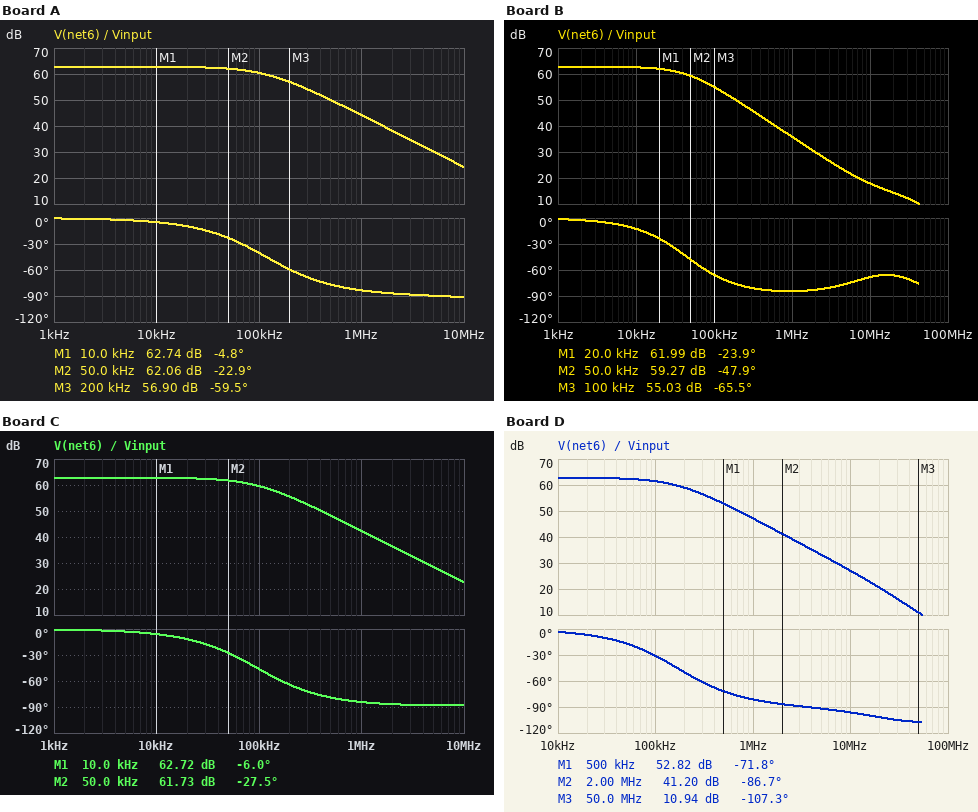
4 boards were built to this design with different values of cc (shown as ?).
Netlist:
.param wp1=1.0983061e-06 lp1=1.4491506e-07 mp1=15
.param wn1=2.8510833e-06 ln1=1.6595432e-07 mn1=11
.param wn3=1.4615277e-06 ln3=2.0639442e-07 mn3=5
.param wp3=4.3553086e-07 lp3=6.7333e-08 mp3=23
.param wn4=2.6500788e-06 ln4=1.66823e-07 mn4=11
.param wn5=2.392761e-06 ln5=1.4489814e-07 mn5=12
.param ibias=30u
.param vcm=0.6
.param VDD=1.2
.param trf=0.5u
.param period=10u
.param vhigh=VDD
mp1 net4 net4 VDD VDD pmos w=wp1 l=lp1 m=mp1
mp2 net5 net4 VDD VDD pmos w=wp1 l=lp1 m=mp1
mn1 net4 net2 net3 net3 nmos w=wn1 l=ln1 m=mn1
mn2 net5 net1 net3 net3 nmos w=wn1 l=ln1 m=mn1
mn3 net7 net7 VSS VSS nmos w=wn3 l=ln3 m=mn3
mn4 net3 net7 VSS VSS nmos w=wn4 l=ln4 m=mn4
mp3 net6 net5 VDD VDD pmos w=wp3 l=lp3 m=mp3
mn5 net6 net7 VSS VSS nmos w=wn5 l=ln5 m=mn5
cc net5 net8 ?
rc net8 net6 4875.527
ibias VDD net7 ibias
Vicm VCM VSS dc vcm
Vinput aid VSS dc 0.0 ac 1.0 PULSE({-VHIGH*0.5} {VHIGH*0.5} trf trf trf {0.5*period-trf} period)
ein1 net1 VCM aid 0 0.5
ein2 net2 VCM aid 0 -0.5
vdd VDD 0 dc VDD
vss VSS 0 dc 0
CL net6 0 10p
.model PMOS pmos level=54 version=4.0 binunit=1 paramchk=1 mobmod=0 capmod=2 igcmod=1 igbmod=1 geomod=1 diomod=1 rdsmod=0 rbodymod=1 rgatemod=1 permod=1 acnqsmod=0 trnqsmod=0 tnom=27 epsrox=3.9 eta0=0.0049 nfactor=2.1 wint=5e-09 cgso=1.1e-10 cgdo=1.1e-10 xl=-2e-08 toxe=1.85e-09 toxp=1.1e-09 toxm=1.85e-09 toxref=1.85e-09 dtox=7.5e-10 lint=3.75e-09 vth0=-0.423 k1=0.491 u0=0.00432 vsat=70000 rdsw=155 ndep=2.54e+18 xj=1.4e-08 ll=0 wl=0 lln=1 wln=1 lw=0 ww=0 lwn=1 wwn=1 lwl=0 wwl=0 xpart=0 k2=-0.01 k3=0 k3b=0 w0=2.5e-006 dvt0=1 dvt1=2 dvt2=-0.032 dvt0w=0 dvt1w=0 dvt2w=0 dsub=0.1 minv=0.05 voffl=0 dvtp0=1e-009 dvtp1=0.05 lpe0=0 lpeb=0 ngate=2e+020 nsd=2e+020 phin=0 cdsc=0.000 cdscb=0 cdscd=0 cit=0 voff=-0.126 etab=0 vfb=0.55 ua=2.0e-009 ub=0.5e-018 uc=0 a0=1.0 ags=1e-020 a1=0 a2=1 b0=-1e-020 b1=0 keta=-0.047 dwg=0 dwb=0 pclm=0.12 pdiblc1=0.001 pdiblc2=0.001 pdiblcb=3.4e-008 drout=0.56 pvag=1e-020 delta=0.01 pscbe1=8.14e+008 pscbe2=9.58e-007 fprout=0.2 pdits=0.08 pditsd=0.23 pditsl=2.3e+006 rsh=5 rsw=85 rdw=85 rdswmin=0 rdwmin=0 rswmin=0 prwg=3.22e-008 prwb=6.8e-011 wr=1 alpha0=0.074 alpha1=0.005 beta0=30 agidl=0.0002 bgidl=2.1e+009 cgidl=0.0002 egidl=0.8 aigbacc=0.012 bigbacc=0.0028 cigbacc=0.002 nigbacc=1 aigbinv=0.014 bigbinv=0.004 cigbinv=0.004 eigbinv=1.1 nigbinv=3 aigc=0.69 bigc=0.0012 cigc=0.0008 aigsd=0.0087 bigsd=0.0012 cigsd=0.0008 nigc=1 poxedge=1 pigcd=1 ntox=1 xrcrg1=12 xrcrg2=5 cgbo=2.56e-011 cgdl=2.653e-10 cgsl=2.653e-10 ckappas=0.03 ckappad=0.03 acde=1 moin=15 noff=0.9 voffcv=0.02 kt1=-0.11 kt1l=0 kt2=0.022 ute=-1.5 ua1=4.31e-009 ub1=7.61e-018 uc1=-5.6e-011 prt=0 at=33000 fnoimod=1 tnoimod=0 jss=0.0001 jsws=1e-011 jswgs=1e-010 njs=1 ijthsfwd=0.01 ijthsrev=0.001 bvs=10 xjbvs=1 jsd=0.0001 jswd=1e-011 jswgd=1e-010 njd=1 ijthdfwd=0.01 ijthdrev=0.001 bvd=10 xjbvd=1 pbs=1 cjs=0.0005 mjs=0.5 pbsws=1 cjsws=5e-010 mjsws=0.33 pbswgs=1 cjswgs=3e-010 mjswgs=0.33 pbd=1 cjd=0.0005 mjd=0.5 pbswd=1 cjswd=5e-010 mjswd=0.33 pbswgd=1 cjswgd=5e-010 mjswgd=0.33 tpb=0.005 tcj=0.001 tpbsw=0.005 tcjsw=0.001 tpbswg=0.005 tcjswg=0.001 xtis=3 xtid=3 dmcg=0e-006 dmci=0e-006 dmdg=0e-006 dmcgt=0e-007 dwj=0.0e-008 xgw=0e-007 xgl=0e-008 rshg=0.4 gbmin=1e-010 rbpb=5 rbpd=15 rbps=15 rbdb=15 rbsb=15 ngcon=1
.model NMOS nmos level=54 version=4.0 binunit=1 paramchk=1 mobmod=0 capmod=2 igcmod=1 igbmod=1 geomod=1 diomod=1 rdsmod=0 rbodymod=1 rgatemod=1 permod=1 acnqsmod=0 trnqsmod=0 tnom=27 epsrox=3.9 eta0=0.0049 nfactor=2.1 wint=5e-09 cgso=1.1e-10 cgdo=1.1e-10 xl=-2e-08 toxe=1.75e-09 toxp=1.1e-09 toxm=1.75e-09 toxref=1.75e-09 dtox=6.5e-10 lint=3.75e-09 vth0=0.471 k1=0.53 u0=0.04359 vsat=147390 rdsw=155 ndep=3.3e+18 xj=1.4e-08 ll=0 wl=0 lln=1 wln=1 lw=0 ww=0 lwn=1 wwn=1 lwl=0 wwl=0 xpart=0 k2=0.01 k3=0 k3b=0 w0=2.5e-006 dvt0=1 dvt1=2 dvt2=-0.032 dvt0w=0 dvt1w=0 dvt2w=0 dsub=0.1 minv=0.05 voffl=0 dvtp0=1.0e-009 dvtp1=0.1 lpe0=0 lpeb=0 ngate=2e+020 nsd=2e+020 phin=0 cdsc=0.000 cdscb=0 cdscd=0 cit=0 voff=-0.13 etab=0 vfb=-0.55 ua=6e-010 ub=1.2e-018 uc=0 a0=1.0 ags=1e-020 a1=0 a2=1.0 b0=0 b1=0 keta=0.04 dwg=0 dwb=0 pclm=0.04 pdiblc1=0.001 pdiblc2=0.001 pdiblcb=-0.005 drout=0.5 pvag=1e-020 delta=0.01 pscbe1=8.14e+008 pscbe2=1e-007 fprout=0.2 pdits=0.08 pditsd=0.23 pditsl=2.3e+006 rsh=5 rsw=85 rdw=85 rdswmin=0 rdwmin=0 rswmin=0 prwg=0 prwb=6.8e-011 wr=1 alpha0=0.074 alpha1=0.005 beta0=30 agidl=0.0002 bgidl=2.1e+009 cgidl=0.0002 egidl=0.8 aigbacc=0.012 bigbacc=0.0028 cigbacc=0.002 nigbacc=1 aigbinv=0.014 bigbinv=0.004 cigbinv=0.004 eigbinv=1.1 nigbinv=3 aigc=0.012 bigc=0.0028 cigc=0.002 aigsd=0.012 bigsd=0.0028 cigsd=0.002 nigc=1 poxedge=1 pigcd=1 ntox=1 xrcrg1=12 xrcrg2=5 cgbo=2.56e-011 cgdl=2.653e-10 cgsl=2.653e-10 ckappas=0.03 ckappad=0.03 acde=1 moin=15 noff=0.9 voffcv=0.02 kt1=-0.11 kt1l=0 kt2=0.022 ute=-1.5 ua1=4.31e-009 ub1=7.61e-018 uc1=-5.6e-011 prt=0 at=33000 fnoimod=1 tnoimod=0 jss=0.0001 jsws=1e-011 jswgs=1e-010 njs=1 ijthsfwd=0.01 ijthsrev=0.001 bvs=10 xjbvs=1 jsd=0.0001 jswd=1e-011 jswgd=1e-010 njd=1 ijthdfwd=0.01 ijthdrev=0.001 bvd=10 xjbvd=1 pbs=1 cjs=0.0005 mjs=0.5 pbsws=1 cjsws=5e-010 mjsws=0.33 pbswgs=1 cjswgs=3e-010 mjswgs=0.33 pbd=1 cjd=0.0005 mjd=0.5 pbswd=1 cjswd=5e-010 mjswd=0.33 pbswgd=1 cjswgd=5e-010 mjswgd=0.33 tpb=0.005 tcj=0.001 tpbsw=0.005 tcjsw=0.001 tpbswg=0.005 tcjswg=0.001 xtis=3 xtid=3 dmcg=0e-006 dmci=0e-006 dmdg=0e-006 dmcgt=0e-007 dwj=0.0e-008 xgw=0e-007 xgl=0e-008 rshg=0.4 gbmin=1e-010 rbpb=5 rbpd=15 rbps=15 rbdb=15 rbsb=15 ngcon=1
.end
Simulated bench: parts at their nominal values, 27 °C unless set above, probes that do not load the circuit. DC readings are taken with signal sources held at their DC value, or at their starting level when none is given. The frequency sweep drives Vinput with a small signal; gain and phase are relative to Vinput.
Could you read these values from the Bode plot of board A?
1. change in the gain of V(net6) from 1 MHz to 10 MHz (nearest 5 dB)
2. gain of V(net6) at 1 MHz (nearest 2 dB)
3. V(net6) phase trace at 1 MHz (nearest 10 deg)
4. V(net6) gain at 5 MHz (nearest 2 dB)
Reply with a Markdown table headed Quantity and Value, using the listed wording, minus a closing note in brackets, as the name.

| Quantity | Value |
|---|---|
| change in the gain of V(net6) from 1 MHz to 10 MHz | -20 dB |
| gain of V(net6) at 1 MHz | 44 dB |
| V(net6) phase trace at 1 MHz | -80 deg |
| V(net6) gain at 5 MHz | 30 dB |
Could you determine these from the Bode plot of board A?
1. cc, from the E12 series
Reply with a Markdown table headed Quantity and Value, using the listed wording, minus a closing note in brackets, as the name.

| Quantity | Value |
|---|---|
| cc, from the E12 series | 1.2 pF |
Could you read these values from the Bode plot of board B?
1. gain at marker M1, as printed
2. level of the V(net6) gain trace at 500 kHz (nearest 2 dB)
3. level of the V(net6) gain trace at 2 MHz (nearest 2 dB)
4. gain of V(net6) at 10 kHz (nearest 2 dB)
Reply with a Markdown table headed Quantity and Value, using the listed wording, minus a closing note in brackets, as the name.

| Quantity | Value |
|---|---|
| gain at marker M1, as printed | 61.99 dB |
| level of the V(net6) gain trace at 500 kHz | 42 dB |
| level of the V(net6) gain trace at 2 MHz | 30 dB |
| gain of V(net6) at 10 kHz | 62 dB |
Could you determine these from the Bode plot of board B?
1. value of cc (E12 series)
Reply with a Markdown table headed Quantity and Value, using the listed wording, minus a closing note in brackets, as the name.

| Quantity | Value |
|---|---|
| value of cc | 3.3 pF |
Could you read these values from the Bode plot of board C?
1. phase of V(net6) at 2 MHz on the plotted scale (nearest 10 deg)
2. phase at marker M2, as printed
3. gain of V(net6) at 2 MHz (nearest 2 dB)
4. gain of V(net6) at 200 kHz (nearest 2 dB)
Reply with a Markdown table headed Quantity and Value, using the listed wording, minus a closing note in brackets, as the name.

| Quantity | Value |
|---|---|
| phase of V(net6) at 2 MHz on the plotted scale | -90 deg |
| phase at marker M2, as printed | -27.5 deg |
| gain of V(net6) at 2 MHz | 36 dB |
| gain of V(net6) at 200 kHz | 56 dB |
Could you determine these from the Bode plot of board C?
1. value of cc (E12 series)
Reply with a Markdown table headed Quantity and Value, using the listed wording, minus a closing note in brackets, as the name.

| Quantity | Value |
|---|---|
| value of cc | 1.5 pF |
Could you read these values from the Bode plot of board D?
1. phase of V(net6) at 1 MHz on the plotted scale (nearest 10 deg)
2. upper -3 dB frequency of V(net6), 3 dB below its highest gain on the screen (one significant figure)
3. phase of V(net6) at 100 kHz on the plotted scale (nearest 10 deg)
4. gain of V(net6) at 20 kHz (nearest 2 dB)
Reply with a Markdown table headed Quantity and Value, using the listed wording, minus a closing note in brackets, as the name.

| Quantity | Value |
|---|---|
| phase of V(net6) at 1 MHz on the plotted scale | -80 deg |
| upper -3 dB frequency of V(net6), 3 dB below its highest gain on the screen | 200 kHz |
| phase of V(net6) at 100 kHz on the plotted scale | -30 deg |
| gain of V(net6) at 20 kHz | 62 dB |
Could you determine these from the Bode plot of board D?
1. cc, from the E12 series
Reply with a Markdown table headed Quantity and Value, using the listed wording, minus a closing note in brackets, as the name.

| Quantity | Value |
|---|---|
| cc, from the E12 series | 820 fF |
